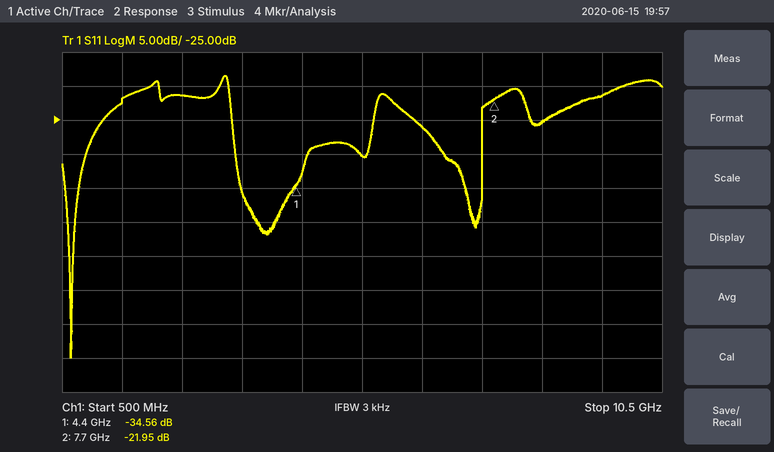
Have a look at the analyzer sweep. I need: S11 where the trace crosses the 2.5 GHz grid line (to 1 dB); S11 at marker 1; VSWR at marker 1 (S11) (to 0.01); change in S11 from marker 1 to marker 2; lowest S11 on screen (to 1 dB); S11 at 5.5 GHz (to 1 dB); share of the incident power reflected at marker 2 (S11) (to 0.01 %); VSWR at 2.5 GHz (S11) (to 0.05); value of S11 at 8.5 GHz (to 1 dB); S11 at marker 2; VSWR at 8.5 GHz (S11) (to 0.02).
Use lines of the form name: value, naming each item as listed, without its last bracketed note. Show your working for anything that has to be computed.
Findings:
S11 where the trace crosses the 2.5 GHz grid line: -21 dB
S11 at marker 1: -34.56 dB
VSWR at marker 1 (S11): (1 + 0.0187)/(1 − 0.0187) ≈ 1.04
change in S11 from marker 1 to marker 2: -21.95 − (-34.56) = 12.61 dB
lowest S11 on screen: -60 dB
S11 at 5.5 GHz: -30 dB
share of the incident power reflected at marker 2 (S11): 10^(-21.95/10) ≈ 0.64 %
VSWR at 2.5 GHz (S11): |Γ| = 10^(-21/20) = 0.0891; VSWR = (1 + 0.0891)/(1 − 0.0891) ≈ 1.20
value of S11 at 8.5 GHz: -25 dB
S11 at marker 2: -21.95 dB
VSWR at 8.5 GHz (S11): |Γ| = 10^(-25/20) = 0.0562; VSWR = (1 + 0.0562)/(1 − 0.0562) ≈ 1.12
